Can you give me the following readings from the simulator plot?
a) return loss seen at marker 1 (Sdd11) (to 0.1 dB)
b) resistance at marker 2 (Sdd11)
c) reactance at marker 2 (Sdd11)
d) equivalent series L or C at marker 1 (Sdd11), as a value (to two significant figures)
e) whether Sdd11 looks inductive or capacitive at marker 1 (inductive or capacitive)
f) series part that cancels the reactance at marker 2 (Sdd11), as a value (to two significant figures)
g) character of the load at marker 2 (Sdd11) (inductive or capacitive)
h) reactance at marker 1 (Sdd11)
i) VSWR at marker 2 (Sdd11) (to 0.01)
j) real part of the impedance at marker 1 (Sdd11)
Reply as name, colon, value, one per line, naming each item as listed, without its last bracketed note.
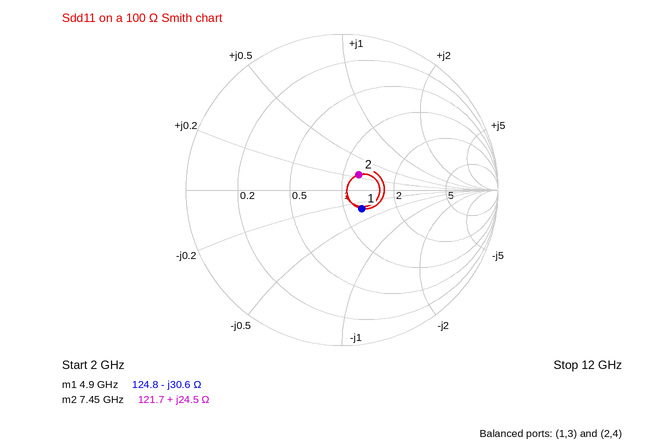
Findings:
return loss seen at marker 1 (Sdd11): 15.2 dB
resistance at marker 2: 121.7 Ω
reactance at marker 2: +24.5 Ω
equivalent series L or C at marker 1 (Sdd11), as a value: 1.1 pF
whether Sdd11 looks inductive or capacitive at marker 1: capacitive
series part that cancels the reactance at marker 2 (Sdd11), as a value: 870 fF
character of the load at marker 2 (Sdd11): inductive
reactance at marker 1: -30.6 Ω
VSWR at marker 2 (Sdd11): 1.34
real part of the impedance at marker 1: 124.8 Ω
